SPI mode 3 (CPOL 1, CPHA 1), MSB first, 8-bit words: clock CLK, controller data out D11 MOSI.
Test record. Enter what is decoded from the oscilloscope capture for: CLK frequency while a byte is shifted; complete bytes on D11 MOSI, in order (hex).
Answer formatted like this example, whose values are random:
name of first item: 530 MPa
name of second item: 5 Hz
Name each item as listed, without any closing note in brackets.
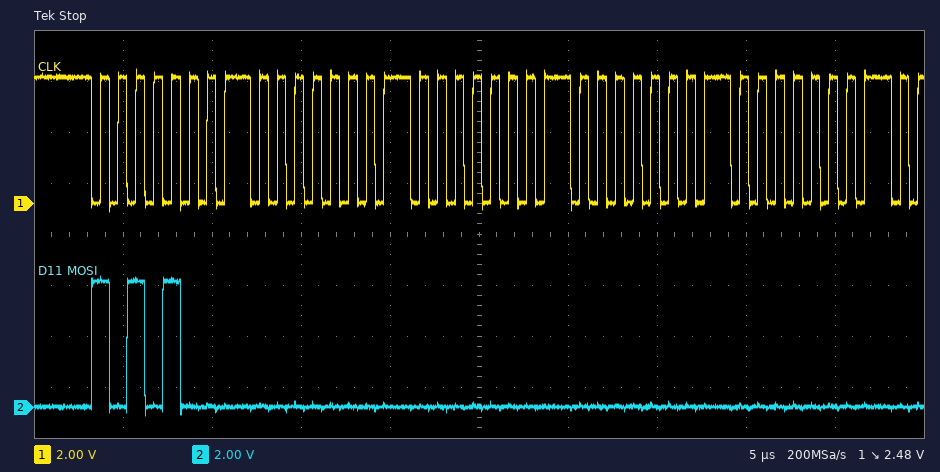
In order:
CLK frequency while a byte is shifted: 1 MHz
complete bytes on D11 MOSI, in order: A8 00 00 00 00
